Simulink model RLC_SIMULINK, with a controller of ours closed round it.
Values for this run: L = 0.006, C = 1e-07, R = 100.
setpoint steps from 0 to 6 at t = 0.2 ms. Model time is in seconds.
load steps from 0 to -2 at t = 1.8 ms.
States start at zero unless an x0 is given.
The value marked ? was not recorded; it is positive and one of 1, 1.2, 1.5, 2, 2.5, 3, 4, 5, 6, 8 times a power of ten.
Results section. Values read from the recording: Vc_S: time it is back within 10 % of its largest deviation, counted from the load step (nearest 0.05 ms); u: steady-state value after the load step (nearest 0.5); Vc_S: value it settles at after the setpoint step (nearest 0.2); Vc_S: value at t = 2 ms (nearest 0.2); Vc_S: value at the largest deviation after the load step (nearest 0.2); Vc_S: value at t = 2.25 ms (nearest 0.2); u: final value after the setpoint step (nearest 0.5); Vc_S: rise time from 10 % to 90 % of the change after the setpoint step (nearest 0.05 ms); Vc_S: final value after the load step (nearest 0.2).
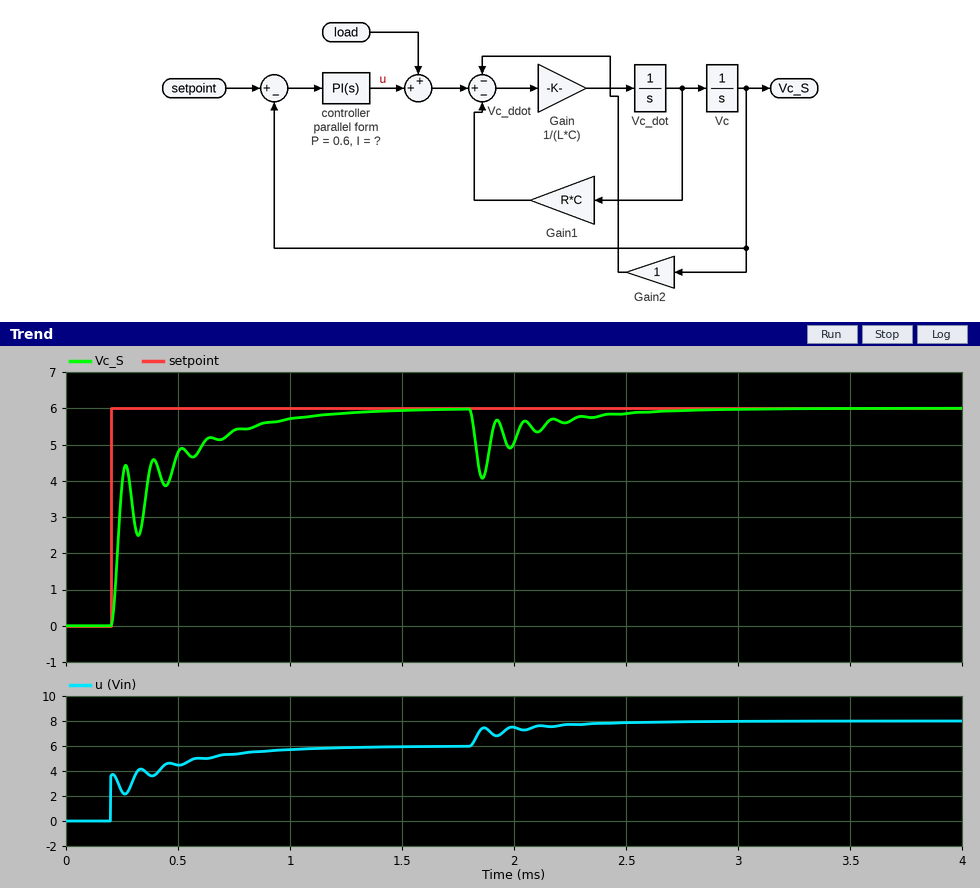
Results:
0.60 ms
8.0
6.0
5.0
4.0
5.6
6.0
0.55 ms
6.0
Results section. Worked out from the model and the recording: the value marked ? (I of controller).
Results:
5000
